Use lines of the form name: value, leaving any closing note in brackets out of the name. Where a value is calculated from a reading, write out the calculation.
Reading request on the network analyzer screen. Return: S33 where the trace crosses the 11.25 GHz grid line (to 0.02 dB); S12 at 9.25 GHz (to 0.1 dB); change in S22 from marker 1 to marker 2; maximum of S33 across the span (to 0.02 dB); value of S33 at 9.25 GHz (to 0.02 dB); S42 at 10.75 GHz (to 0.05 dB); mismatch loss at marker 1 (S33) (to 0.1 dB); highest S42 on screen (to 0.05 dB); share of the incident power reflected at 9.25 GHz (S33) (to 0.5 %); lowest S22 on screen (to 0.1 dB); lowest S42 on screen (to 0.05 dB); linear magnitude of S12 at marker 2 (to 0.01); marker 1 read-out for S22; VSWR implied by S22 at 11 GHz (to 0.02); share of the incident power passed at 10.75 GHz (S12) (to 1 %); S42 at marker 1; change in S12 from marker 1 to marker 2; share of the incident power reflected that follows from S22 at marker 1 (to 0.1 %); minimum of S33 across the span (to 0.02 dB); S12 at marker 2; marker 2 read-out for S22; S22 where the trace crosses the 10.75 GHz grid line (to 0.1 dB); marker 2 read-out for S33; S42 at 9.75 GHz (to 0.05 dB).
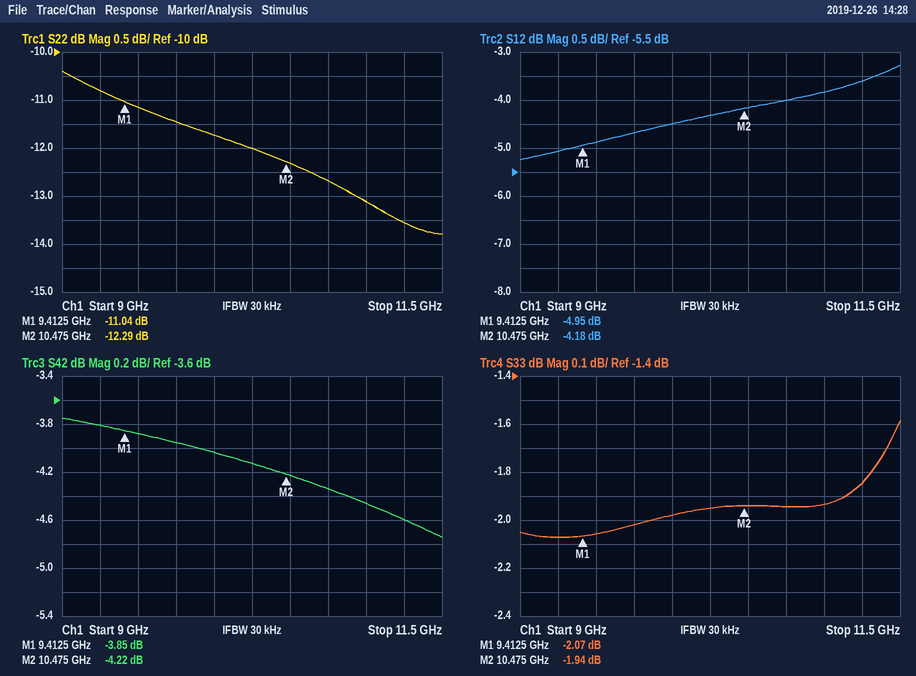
S33 where the trace crosses the 11.25 GHz grid line: -1.84 dB
S12 at 9.25 GHz: -5.1 dB
change in S22 from marker 1 to marker 2: -12.29 − (-11.04) = -1.25 dB
maximum of S33 across the span: -1.58 dB
value of S33 at 9.25 GHz: -2.08 dB
S42 at 10.75 GHz: -4.35 dB
mismatch loss at marker 1 (S33): −10 log10(1 − 10^(-2.07/10)) ≈ 4.2 dB
highest S42 on screen: -3.75 dB
share of the incident power reflected at 9.25 GHz (S33): 10^(-2.08/10) ≈ 61.9 %, so 62.0 % to the nearest 0.5 %
lowest S22 on screen: -13.8 dB
lowest S42 on screen: -4.75 dB
linear magnitude of S12 at marker 2: 10^(-4.18/20) ≈ 0.62
marker 1 read-out for S22: -11.04 dB
VSWR implied by S22 at 11 GHz: |Γ| = 10^(-13.1/20) = 0.2213; VSWR = (1 + 0.2213)/(1 − 0.2213) ≈ 1.57, so 1.56 to the nearest 0.02
share of the incident power passed at 10.75 GHz (S12): 10^(-4/10) ≈ 40 %
S42 at marker 1: -3.85 dB
change in S12 from marker 1 to marker 2: -4.18 − (-4.95) = 0.77 dB
share of the incident power reflected that follows from S22 at marker 1: 10^(-11.04/10) ≈ 7.9 %
minimum of S33 across the span: -2.08 dB
S12 at marker 2: -4.18 dB
marker 2 read-out for S22: -12.29 dB
S22 where the trace crosses the 10.75 GHz grid line: -12.7 dB
marker 2 read-out for S33: -1.94 dB
S42 at 9.75 GHz: -3.95 dB
